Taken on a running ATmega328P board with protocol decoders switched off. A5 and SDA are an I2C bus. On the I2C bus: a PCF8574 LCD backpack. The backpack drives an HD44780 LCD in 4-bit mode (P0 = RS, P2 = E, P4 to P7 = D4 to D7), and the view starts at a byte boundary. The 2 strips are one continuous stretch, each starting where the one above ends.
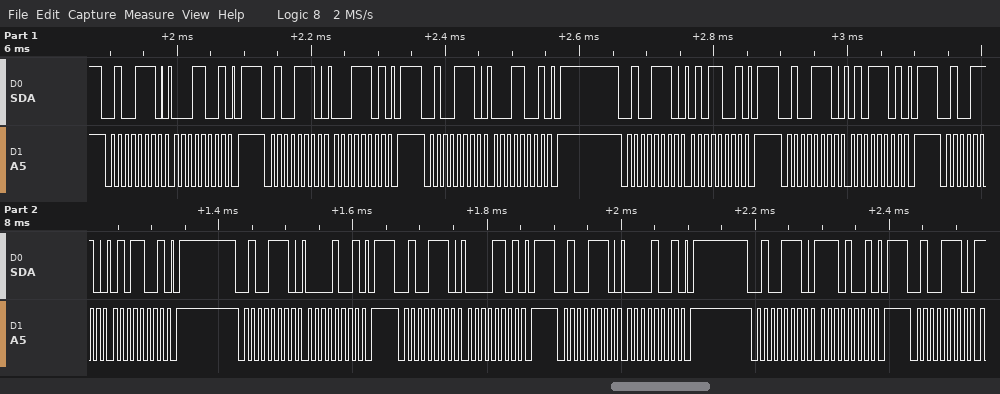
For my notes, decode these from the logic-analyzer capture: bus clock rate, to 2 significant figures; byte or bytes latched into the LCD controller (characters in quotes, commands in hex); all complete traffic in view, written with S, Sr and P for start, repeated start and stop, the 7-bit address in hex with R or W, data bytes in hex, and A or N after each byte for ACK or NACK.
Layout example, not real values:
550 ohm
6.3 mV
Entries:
100 kHz
data 0x15
S 27W A 19 A P S 27W A 1D A P S 27W A 19 A P S 27W A 59 A P S 27W A 5D A P S 27W A 59 A P S 27W A 09 A P S 27W A 0D A P S 27W A 09 A P S 27W A E9 A P S 27W A
